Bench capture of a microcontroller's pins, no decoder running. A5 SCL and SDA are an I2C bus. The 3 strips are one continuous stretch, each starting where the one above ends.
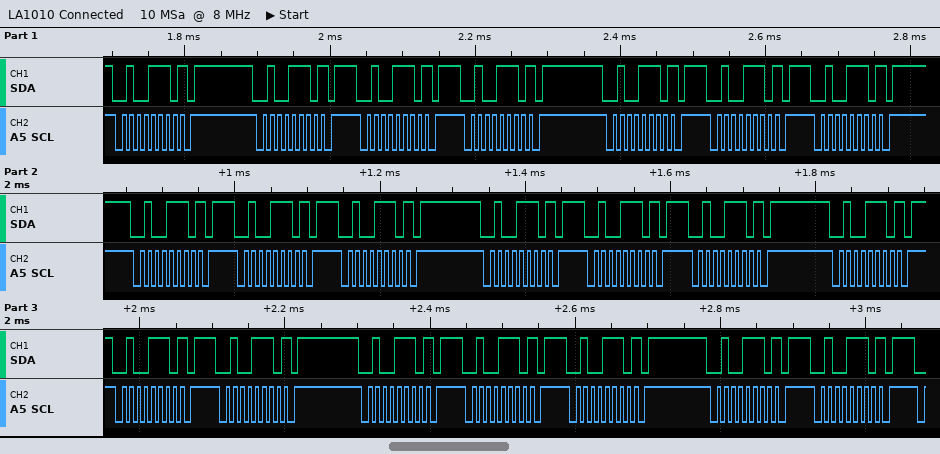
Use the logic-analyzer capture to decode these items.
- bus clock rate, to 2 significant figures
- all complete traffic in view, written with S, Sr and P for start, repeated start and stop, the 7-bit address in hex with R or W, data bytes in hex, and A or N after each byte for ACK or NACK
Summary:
100 kHz
S 27W N P S 27W N P S 27W N P S 27W N P S 27W N P S 27W N P S 27W N P S 27W N P S 27W N P S 27W N P S 27W N P S 27W N P S 27W N P S 27W N P S 27W N P S 27W N P S 27W N P S 27W N P S 27W N P S 27W N P S 27W N P
